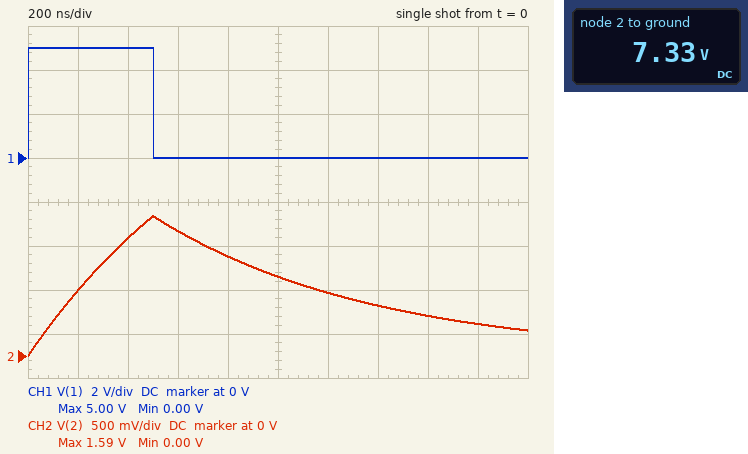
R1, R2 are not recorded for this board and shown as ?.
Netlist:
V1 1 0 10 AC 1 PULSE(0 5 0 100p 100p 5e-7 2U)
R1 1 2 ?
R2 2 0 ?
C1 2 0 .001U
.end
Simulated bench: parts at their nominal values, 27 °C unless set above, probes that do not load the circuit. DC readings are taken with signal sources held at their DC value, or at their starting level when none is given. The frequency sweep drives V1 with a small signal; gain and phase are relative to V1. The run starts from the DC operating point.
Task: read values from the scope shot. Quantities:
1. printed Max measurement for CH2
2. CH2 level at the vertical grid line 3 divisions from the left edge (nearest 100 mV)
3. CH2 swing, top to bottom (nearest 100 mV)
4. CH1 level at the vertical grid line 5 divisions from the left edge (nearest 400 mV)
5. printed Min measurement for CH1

1.59 V
1.4 V
1.6 V
0 V
0.00 V
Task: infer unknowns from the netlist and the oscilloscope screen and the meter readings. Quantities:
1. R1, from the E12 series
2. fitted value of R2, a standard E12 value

1.2 kΩ
3.3 kΩ
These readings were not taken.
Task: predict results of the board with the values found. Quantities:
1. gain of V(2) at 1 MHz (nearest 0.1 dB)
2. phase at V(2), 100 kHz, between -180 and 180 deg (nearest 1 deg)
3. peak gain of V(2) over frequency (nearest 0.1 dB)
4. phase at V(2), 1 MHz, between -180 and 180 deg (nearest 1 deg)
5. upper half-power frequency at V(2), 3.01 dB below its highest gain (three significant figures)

-17.7 dB
-29 deg
-2.7 dB
-80 deg
181 kHz
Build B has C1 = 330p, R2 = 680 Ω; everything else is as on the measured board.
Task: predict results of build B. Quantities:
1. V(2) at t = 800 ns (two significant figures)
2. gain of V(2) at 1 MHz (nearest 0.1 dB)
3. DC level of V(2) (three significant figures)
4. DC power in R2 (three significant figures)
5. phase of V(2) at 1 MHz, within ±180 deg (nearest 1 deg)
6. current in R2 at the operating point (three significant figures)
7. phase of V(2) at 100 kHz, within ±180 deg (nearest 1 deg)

220 mV
-11.4 dB
3.62 V
19.2 mW
-42 deg
5.32 mA
-5 deg
